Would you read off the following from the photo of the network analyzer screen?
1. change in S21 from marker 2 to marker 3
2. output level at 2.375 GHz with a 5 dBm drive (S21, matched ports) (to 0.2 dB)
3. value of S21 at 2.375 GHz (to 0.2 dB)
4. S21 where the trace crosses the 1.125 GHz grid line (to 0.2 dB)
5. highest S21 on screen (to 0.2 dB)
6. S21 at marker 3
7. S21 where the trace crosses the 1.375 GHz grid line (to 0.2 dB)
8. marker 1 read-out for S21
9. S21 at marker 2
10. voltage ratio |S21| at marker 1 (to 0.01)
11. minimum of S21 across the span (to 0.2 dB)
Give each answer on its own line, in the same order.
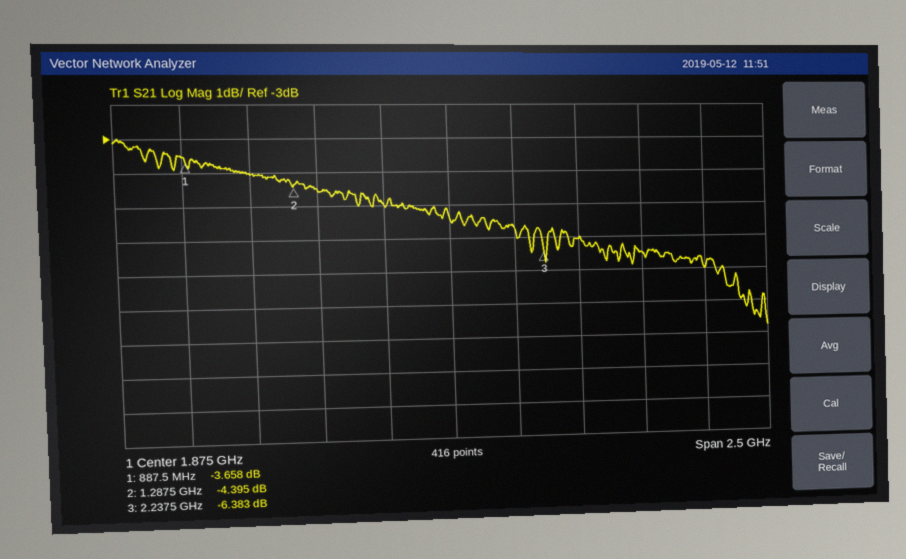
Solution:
-1.988 dB
-1.0 dBm
-6.0 dB
-4.0 dB
-3.0 dB
-6.383 dB
-4.4 dB
-3.658 dB
-4.395 dB
0.66
-8.8 dB
